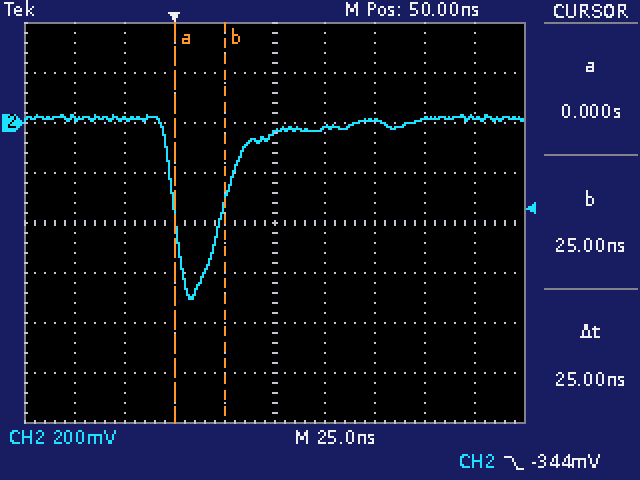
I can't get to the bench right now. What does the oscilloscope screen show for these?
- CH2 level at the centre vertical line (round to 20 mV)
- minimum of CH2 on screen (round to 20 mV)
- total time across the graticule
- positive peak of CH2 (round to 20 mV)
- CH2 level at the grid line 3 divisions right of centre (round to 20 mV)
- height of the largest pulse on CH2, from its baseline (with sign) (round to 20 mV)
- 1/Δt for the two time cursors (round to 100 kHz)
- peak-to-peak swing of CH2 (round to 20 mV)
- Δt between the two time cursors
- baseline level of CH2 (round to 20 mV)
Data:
-40 mV
-700 mV
250 ns
40 mV
20 mV
-720 mV
40.0 MHz
740 mV
25 ns
20 mV
